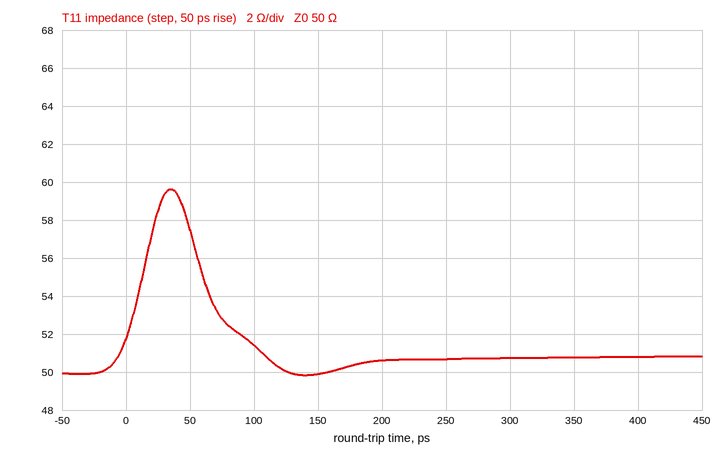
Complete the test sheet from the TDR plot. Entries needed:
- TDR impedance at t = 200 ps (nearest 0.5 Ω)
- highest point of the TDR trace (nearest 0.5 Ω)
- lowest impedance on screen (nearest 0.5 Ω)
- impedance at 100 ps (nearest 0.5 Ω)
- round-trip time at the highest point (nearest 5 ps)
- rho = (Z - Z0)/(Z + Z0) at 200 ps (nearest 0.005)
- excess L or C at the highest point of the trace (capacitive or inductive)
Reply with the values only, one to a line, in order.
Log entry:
50.5 Ω
59.5 Ω
50.0 Ω
51.5 Ω
35 ps
+0.005
inductive
